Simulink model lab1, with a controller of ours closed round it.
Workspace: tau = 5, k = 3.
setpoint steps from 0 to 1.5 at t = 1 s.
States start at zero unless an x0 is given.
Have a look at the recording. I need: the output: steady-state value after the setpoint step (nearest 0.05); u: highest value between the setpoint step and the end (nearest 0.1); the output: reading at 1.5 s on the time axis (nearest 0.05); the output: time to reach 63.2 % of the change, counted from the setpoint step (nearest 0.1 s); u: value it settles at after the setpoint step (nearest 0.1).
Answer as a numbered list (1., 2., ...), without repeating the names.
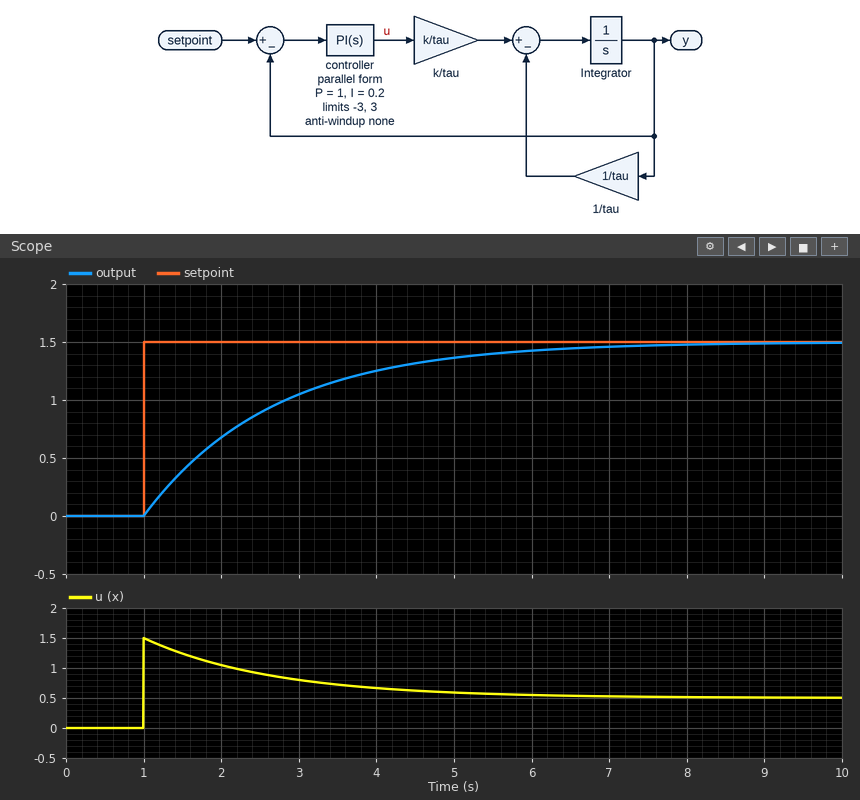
1. 1.50
2. 1.5
3. 0.40
4. 1.7 s
5. 0.5
